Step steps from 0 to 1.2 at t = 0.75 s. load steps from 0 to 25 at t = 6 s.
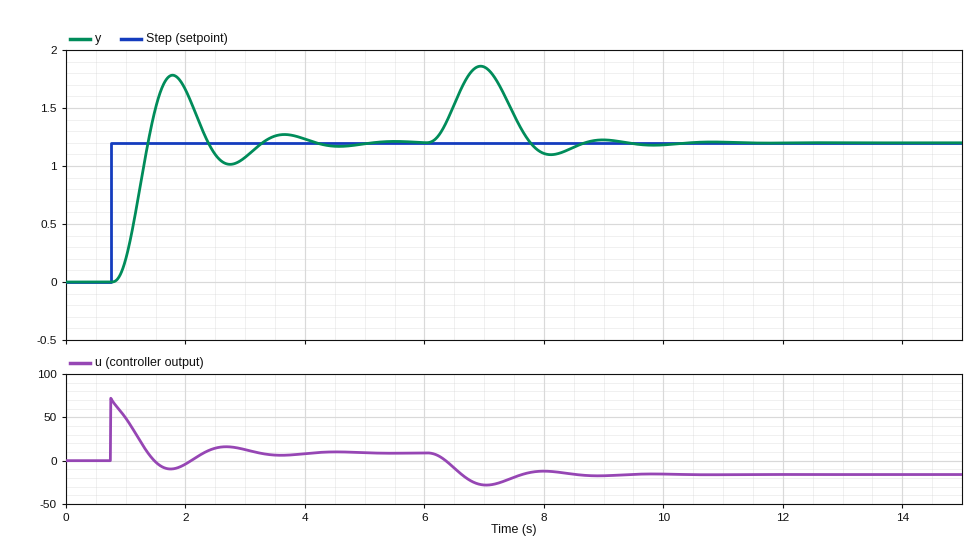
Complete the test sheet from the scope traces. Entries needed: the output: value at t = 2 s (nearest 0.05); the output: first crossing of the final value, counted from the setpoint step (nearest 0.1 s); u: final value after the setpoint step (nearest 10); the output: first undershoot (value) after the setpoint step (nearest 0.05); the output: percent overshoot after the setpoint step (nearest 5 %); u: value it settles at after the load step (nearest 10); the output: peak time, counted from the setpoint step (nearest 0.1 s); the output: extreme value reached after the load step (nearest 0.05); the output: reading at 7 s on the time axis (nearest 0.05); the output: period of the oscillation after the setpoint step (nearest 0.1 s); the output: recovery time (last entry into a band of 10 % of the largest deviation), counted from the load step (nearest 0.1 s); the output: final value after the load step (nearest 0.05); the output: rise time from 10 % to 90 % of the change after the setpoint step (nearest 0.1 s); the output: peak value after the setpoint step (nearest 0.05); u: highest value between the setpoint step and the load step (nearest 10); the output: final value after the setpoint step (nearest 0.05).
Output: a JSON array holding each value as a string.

["1.65", "0.6 s", "10", "1.00", "50 %", "-20", "1.0 s", "1.85", "1.85", "1.9 s", "2.4 s", "1.20", "0.4 s", "1.80", "70", "1.20"]
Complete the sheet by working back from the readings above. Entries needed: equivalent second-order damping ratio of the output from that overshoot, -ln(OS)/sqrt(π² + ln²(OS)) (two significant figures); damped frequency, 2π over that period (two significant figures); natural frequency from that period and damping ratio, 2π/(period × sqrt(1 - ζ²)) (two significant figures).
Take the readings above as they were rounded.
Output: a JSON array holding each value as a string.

["0.22", "3.3 rad/s", "3.4 rad/s"]
